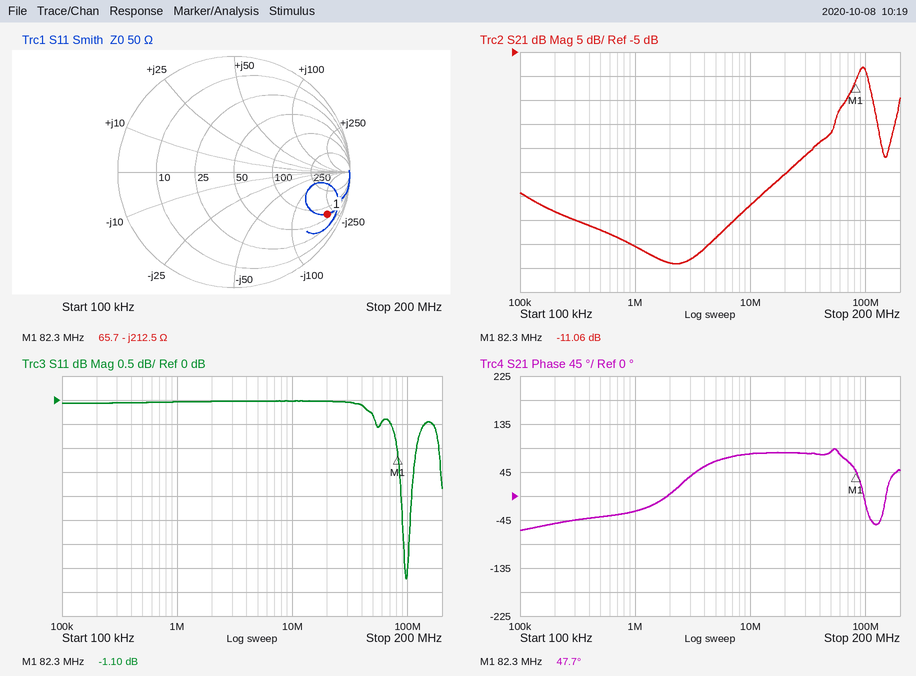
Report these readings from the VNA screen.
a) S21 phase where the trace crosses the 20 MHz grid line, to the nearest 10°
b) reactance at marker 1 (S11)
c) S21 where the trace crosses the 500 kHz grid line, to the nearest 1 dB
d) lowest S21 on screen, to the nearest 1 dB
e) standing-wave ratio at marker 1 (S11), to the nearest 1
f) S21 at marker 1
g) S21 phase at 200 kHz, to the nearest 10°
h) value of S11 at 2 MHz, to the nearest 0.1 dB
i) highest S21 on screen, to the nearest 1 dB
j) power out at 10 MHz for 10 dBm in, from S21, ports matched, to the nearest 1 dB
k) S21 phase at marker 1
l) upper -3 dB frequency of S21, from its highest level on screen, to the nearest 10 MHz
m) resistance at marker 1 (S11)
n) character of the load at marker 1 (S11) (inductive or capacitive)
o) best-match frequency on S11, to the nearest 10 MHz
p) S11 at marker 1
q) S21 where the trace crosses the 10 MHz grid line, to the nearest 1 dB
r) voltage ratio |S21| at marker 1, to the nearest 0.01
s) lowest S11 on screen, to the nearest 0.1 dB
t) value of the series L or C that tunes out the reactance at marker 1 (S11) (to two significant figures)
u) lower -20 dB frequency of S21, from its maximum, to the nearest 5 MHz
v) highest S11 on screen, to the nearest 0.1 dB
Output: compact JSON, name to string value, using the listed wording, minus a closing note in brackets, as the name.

{"S21 phase where the trace crosses the 20 MHz grid line, to the nearest 10°": "80°", "reactance at marker 1": "-212.5 Ω", "S21 where the trace crosses the 500 kHz grid line, to the nearest 1 dB": "-42 dB", "lowest S21 on screen, to the nearest 1 dB": "-49 dB", "standing-wave ratio at marker 1 (S11), to the nearest 1": "16", "S21 at marker 1": "-11.06 dB", "S21 phase at 200 kHz, to the nearest 10°": "-50°", "value of S11 at 2 MHz, to the nearest 0.1 dB": "0.0 dB", "highest S21 on screen, to the nearest 1 dB": "-8 dB", "power out at 10 MHz for 10 dBm in, from S21, ports matched, to the nearest 1 dB": "-27 dBm", "S21 phase at marker 1": "47.7°", "upper -3 dB frequency of S21, from its highest level on screen, to the nearest 10 MHz": "110 MHz", "resistance at marker 1": "65.7 Ω", "character of the load at marker 1 (S11)": "capacitive", "best-match frequency on S11, to the nearest 10 MHz": "100 MHz", "S11 at marker 1": "-1.10 dB", "S21 where the trace crosses the 10 MHz grid line, to the nearest 1 dB": "-37 dB", "voltage ratio |S21| at marker 1, to the nearest 0.01": "0.28", "lowest S11 on screen, to the nearest 0.1 dB": "-3.7 dB", "value of the series L or C that tunes out the reactance at marker 1 (S11)": "410 nH", "lower -20 dB frequency of S21, from its maximum, to the nearest 5 MHz": "25 MHz", "highest S11 on screen, to the nearest 0.1 dB": "0.0 dB"}
